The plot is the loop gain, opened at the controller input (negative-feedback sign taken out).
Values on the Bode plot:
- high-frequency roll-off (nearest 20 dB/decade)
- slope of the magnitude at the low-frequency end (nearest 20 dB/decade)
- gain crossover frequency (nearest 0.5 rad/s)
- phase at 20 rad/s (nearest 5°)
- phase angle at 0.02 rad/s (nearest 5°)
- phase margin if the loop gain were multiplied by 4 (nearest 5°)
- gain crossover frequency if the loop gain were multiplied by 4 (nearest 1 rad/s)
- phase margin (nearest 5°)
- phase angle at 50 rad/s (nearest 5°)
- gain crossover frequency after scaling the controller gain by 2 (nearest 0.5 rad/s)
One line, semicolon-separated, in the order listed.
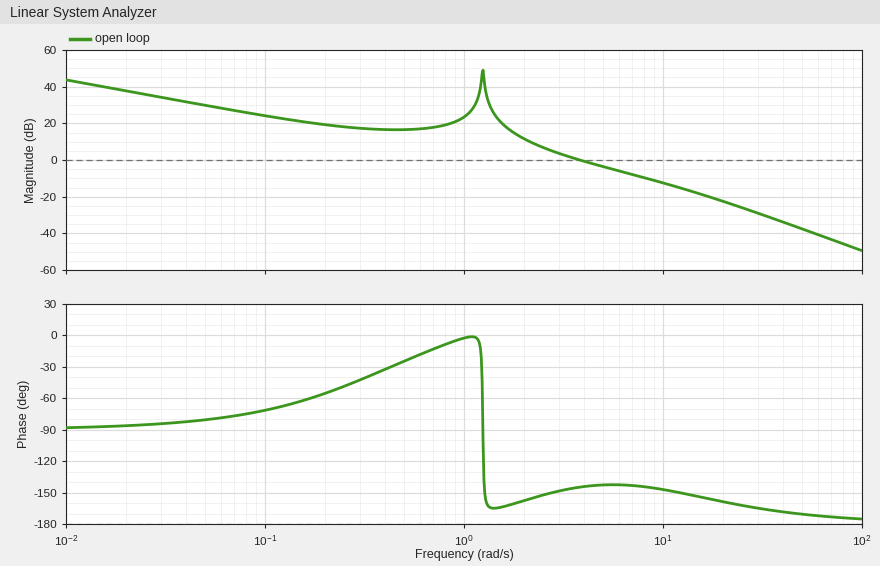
-40 dB/decade; -20 dB/decade; 4.0 rad/s; -160°; -85°; 35°; 10 rad/s; 35°; -170°; 6.0 rad/s
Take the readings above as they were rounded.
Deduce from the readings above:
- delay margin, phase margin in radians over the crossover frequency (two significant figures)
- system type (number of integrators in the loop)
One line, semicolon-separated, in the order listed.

0.15 s; 1
